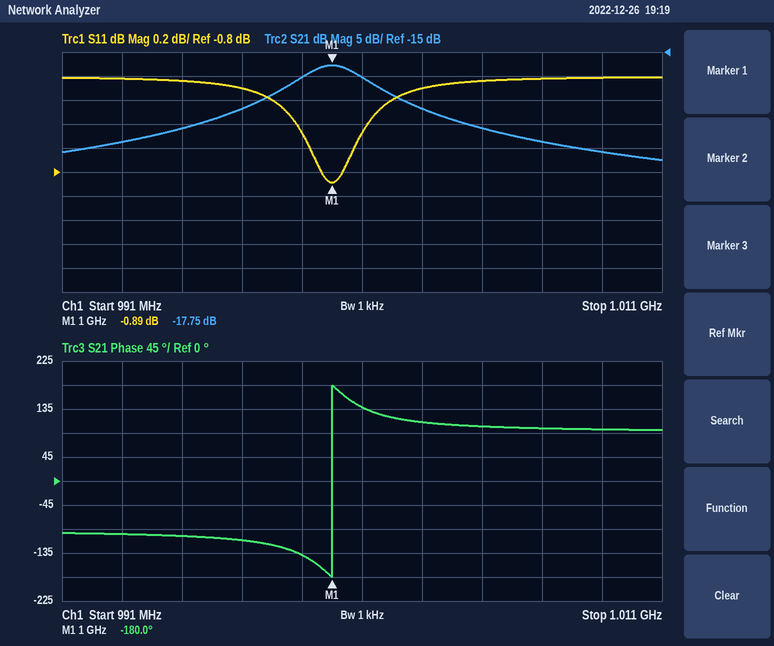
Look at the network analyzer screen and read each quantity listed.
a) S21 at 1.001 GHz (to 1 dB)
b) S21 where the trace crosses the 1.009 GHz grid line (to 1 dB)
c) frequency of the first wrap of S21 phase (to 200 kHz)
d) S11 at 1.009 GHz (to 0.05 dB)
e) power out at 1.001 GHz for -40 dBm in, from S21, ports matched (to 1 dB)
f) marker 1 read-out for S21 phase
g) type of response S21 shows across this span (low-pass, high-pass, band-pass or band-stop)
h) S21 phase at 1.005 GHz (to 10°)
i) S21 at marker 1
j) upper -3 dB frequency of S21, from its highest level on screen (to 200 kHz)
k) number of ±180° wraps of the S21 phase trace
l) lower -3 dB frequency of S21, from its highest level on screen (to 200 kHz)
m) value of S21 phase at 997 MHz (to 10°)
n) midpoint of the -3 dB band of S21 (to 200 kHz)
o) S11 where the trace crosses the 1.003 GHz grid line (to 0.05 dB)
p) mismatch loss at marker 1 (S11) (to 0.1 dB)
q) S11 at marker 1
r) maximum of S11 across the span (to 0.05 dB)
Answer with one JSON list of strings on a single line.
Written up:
["-20 dB", "-36 dB", "1.0000 GHz", "0.00 dB", "-60 dBm", "-180.0°", "band-pass", "100°", "-17.75 dB", "1.0012 GHz", "1", "998.8 MHz", "-110°", "1.0000 GHz", "-0.10 dB", "7.3 dB", "-0.89 dB", "0.00 dB"]
